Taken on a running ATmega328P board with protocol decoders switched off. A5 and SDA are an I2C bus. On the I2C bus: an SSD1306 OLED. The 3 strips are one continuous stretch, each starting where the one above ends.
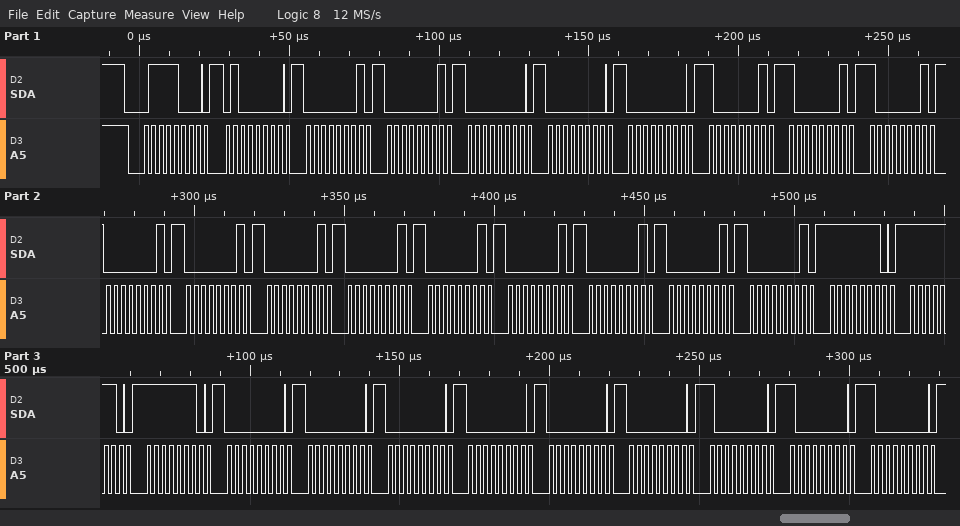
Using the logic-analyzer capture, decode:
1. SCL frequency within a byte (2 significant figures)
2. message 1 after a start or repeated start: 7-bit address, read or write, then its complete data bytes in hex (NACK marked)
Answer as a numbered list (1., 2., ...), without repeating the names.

1. 400 kHz
2. 0x3C write: 40 01 01 00 00 00 81 81 81 01 01 01 01 01 01 01 01 01 FE FE FE 00 00 00 00 00 00 80 80 80
